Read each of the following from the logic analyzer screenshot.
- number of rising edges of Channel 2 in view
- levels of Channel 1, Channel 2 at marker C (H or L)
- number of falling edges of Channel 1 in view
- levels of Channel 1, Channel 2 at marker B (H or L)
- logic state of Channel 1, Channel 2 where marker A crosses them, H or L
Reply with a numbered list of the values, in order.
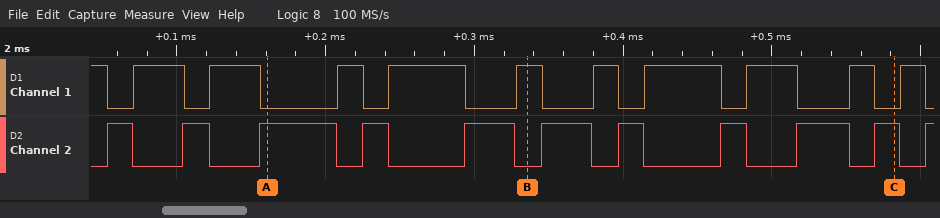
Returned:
1. 11
2. Channel 1=L, Channel 2=H
3. 11
4. Channel 1=H, Channel 2=L
5. Channel 1=L, Channel 2=H
